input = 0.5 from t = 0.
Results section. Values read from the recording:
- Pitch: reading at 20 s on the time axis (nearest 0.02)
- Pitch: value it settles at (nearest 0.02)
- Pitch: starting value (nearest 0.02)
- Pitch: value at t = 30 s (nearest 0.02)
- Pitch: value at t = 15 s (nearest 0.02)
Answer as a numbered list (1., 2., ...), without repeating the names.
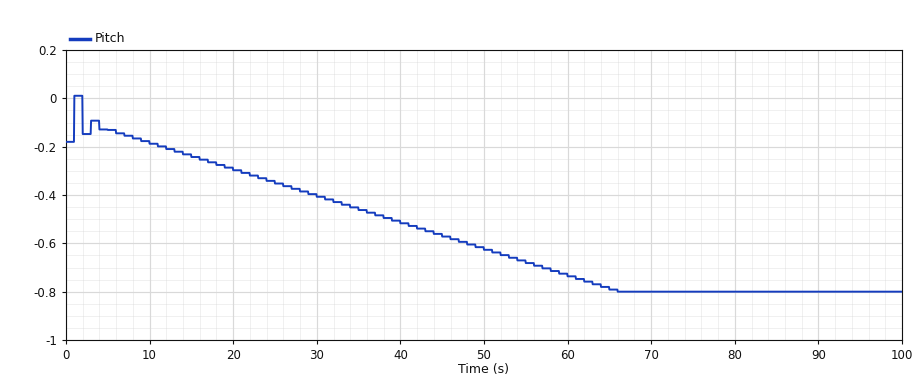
1. -0.30
2. -0.80
3. -0.18
4. -0.40
5. -0.24
